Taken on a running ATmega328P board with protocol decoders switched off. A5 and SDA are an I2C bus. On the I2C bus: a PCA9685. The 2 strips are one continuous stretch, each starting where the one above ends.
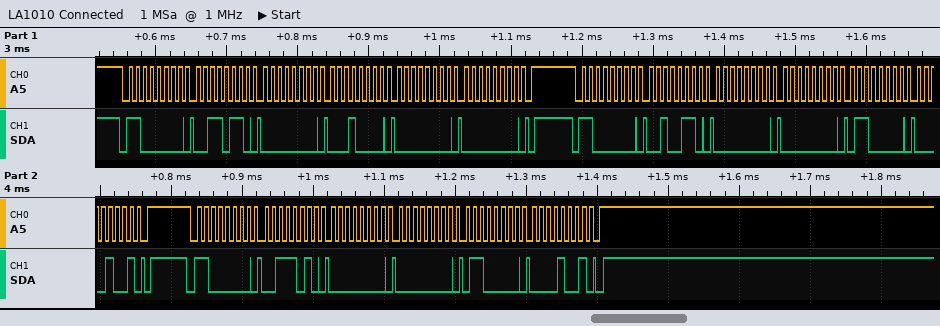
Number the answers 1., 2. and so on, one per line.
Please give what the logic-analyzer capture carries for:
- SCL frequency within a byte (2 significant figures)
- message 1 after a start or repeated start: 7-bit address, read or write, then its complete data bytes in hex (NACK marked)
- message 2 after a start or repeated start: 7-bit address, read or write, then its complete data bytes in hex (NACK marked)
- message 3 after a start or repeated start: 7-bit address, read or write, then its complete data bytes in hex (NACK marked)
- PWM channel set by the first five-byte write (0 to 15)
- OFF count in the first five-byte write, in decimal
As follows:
1. 100 kHz
2. 0x60 write: 36 00 10 00 00
3. 0x60 write: 26 00 00 60 09
4. 0x60 write: 3A 00 00 60 09
5. 12
6. 0
